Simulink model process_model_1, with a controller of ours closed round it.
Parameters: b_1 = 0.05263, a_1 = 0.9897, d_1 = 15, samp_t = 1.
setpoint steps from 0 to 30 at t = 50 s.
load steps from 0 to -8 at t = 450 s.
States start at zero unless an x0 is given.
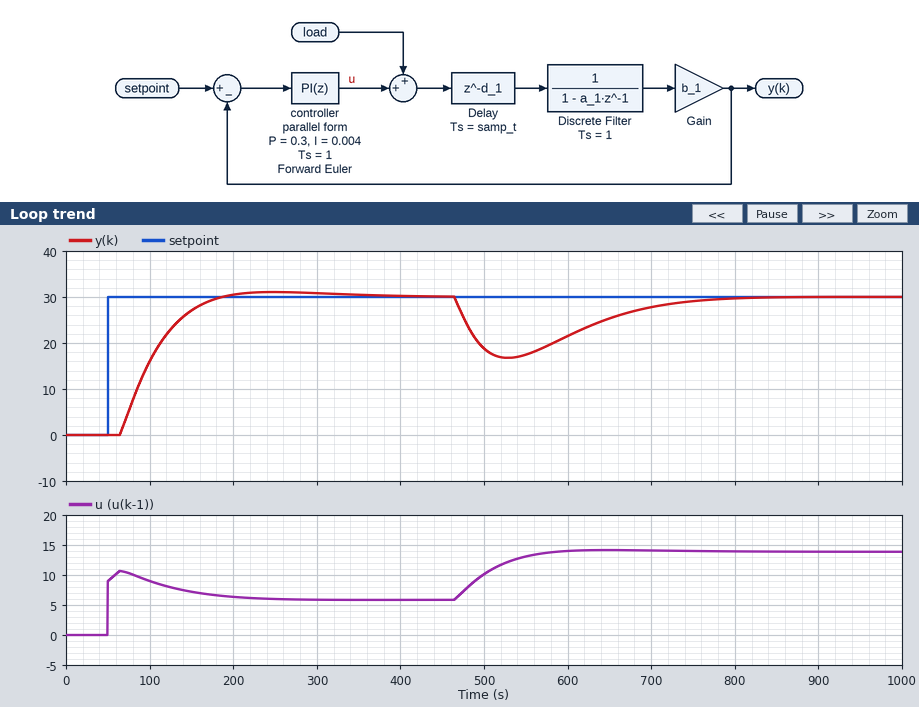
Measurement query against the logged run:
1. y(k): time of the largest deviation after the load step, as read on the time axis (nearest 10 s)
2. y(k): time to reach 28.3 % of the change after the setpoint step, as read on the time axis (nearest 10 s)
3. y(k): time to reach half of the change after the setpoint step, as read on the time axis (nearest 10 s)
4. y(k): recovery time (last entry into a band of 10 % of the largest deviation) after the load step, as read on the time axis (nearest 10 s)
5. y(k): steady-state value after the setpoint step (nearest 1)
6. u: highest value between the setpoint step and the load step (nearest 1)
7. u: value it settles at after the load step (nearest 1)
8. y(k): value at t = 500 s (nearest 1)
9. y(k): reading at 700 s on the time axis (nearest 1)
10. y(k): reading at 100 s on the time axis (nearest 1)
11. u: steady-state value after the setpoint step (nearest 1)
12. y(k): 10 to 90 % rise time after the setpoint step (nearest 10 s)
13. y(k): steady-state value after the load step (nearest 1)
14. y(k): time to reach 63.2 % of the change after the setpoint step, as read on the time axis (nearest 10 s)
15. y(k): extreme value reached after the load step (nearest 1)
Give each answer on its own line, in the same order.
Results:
530 s
80 s
100 s
730 s
30
11
14
19
28
16
6
80 s
30
110 s
17
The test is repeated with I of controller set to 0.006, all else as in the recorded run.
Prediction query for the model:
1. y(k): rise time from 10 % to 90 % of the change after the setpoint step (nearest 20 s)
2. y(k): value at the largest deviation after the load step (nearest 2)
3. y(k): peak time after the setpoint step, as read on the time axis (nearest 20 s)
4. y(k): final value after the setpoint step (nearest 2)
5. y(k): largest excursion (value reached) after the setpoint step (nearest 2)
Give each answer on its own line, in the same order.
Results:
60 s
18
200 s
30
34
